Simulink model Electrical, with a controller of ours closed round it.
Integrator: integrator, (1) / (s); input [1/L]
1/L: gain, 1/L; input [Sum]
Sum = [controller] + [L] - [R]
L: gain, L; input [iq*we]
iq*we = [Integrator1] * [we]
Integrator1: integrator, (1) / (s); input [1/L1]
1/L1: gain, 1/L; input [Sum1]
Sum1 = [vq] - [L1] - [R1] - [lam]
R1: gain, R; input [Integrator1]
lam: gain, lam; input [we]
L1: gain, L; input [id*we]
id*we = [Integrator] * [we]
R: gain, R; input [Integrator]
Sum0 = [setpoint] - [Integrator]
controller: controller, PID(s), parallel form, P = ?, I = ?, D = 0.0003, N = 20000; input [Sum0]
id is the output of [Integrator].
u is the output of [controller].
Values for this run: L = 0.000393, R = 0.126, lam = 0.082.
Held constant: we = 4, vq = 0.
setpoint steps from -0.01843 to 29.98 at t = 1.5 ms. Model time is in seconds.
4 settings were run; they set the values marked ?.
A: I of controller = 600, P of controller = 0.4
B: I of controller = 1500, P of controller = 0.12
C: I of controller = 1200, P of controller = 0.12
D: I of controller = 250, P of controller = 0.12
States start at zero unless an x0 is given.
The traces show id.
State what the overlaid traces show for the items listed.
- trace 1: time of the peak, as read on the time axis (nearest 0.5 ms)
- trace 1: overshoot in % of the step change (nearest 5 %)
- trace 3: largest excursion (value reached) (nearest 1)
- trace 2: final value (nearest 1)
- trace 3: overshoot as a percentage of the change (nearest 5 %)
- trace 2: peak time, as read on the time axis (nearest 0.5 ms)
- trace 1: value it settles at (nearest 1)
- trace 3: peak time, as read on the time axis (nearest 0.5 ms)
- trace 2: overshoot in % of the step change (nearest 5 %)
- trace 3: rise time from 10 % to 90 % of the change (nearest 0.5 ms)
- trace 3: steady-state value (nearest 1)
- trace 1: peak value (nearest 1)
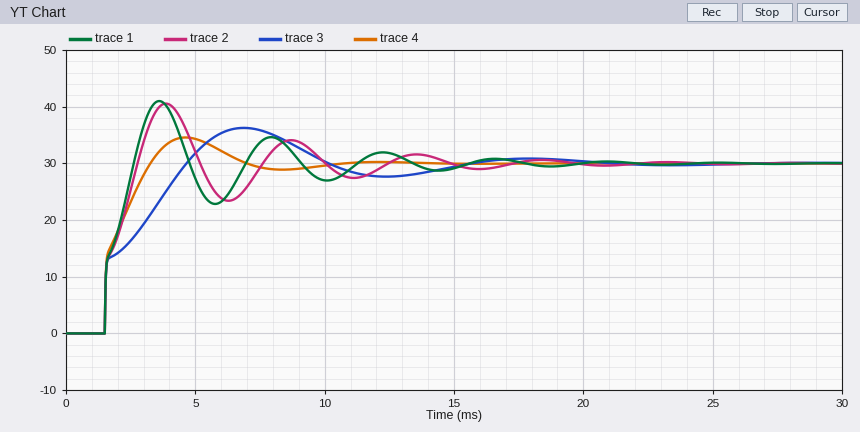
3.5 ms
35 %
36
30
20 %
4.0 ms
30
7.0 ms
35 %
2.5 ms
30
41
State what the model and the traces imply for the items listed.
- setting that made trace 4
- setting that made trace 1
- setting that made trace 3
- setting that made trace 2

A
B
D
C
